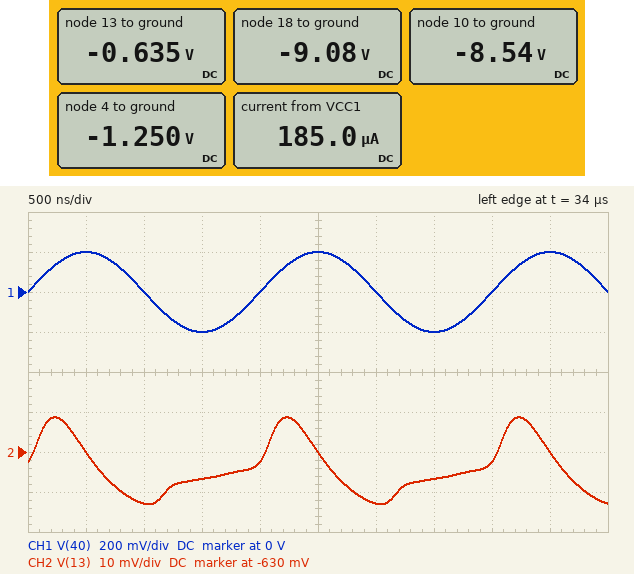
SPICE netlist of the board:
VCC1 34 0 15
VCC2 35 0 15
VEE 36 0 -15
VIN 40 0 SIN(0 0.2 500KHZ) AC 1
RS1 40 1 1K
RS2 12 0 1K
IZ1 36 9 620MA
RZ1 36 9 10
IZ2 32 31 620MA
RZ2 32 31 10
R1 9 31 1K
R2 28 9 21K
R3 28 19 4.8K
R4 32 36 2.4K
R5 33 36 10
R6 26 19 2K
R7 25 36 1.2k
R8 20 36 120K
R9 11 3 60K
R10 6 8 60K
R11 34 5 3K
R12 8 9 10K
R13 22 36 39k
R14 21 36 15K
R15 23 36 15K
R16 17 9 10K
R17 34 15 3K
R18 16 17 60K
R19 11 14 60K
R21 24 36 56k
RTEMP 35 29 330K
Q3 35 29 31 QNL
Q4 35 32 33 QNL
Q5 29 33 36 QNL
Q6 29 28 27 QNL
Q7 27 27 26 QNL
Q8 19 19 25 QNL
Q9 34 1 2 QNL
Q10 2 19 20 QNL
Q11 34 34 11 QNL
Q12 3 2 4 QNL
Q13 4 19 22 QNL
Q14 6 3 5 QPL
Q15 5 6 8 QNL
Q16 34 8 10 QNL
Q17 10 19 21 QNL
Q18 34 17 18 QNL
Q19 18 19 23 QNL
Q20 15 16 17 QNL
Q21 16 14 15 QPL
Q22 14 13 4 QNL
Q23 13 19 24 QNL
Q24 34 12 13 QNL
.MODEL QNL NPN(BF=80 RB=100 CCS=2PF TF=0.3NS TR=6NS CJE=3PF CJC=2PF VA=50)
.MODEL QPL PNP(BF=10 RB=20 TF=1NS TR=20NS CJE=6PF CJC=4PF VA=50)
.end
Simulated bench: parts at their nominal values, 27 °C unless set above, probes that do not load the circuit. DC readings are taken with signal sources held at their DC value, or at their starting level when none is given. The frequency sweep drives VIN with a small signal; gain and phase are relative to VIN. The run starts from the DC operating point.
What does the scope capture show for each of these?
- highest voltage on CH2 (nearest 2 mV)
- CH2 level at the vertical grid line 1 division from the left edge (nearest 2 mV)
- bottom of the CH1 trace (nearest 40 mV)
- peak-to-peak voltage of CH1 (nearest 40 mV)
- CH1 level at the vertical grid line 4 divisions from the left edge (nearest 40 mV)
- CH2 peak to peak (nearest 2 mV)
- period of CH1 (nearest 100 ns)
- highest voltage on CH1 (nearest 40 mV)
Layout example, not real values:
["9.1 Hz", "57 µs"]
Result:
["-622 mV", "-630 mV", "-200 mV", "400 mV", "0 V", "22 mV", "2.0 µs", "200 mV"]
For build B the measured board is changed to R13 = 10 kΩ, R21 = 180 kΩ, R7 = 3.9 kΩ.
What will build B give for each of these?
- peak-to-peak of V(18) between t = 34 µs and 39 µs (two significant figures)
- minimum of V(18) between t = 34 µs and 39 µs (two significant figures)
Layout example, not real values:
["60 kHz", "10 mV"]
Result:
["7.2 V", "-5.5 V"]
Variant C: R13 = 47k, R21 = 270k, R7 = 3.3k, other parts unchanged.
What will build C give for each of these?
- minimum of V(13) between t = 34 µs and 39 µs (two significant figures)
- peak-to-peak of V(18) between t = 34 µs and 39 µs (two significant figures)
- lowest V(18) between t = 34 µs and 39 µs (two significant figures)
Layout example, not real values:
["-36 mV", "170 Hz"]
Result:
["-630 mV", "1.7 V", "-9.1 V"]
